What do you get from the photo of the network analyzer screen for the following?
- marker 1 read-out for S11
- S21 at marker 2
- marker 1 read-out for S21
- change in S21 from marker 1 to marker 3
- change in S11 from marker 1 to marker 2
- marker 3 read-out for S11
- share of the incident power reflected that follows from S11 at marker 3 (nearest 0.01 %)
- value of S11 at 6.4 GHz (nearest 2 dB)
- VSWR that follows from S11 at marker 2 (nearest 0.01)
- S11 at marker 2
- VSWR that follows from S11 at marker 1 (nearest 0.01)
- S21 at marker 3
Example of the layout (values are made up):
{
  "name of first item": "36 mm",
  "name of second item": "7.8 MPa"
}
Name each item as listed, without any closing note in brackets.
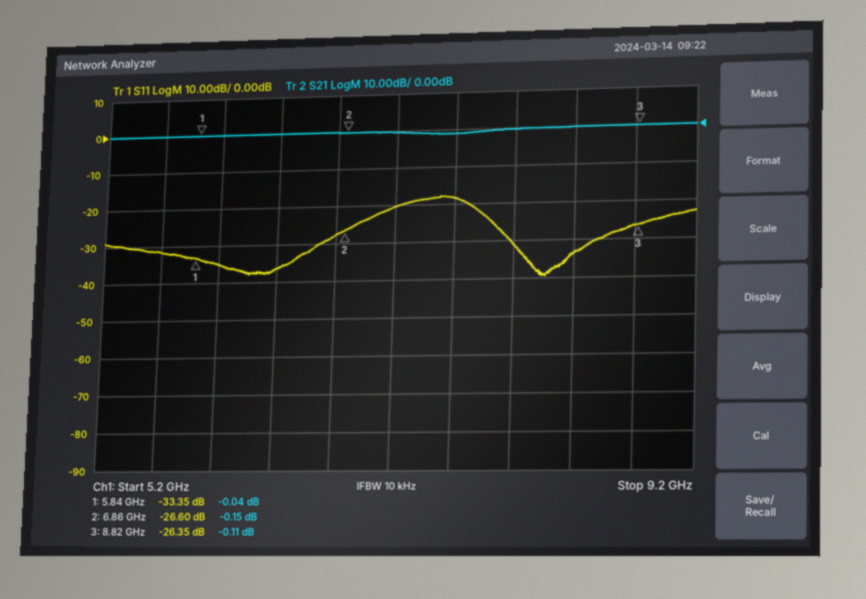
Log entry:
{
  "marker 1 read-out for S11": "-33.35 dB",
  "S21 at marker 2": "-0.15 dB",
  "marker 1 read-out for S21": "-0.04 dB",
  "change in S21 from marker 1 to marker 3": "-0.07 dB",
  "change in S11 from marker 1 to marker 2": "6.75 dB",
  "marker 3 read-out for S11": "-26.35 dB",
  "share of the incident power reflected that follows from S11 at marker 3": "0.23 %",
  "value of S11 at 6.4 GHz": "-36 dB",
  "VSWR that follows from S11 at marker 2": "1.10",
  "S11 at marker 2": "-26.60 dB",
  "VSWR that follows from S11 at marker 1": "1.04",
  "S21 at marker 3": "-0.11 dB"
}
